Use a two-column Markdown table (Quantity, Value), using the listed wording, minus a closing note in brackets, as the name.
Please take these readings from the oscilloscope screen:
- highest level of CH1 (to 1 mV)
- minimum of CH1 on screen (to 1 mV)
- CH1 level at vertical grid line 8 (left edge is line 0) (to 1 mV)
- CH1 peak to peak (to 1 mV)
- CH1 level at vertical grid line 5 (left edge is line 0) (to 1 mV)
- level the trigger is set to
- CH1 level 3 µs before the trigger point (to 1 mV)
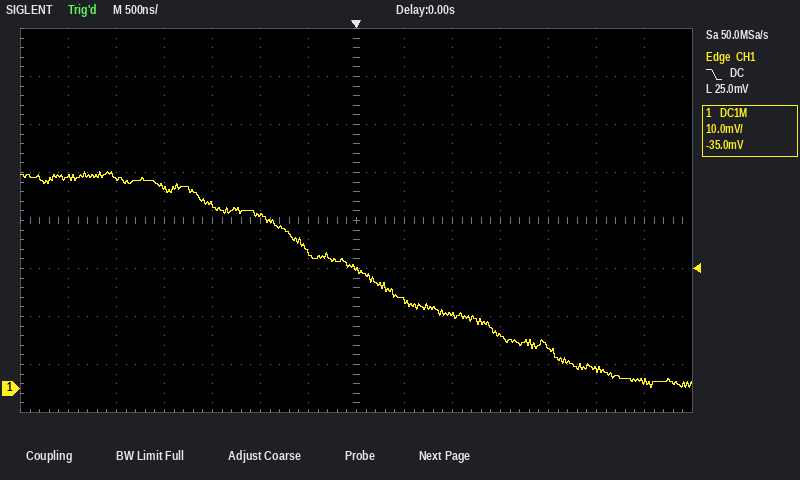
| Quantity | Value |
|---|---|
| highest level of CH1 | 45 mV |
| minimum of CH1 on screen | 0 mV |
| CH1 level at vertical grid line 8 (left edge is line 0) | 18 mV |
| CH1 peak to peak | 45 mV |
| CH1 level at vertical grid line 5 (left edge is line 0) | 36 mV |
| level the trigger is set to | 25.0 mV |
| CH1 level 3 µs before the trigger point | 44 mV |
